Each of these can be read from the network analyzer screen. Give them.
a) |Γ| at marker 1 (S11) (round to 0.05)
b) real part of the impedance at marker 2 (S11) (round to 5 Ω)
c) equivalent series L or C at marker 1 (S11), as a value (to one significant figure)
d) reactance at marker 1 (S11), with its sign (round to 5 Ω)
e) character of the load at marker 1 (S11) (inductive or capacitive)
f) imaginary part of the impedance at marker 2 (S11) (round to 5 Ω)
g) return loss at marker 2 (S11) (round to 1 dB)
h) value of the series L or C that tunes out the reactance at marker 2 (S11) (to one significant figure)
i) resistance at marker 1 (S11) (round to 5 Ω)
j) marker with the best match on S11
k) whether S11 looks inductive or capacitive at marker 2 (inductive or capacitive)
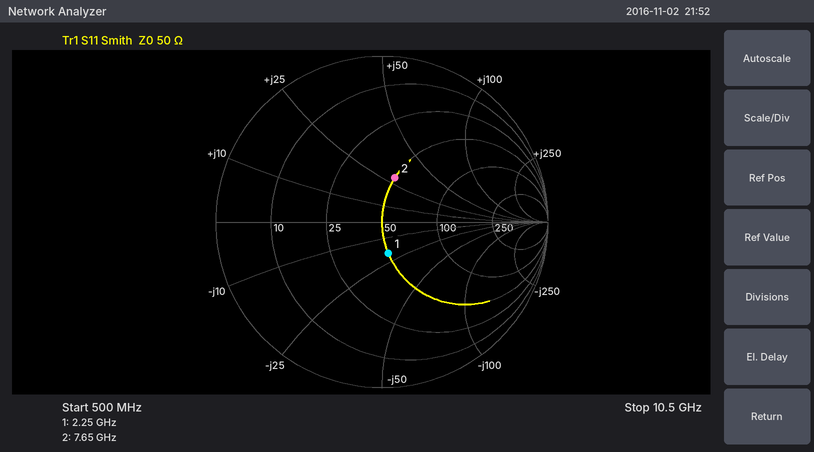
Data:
0.20
50 Ω
4 pF
-20 Ω
capacitive
+30 Ω
11 dB
700 fF
50 Ω
marker 1
inductive
